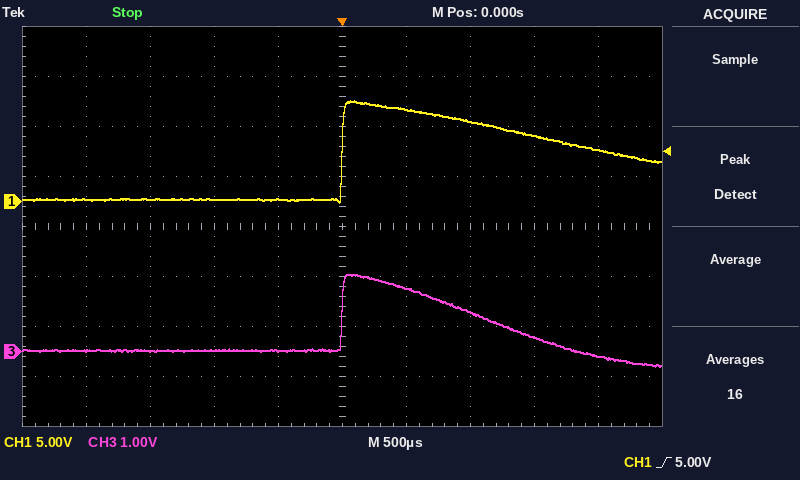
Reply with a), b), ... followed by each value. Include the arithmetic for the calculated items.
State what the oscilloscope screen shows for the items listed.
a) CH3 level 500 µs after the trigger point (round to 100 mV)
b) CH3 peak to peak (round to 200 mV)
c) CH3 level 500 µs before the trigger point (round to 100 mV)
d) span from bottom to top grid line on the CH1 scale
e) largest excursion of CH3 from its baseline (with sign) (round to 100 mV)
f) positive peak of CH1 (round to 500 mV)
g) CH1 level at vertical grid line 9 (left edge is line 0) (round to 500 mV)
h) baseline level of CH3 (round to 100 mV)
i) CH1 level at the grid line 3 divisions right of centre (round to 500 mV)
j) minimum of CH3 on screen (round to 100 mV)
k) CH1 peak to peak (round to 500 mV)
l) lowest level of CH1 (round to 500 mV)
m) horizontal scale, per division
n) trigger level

a) 1.3 V
b) 1.8 V
c) 0.0 V
d) 40 V
e) +1.5 V
f) 10.0 V
g) 5.0 V
h) 0.0 V
i) 6.5 V
j) -300 mV
k) 10.0 V − (0.0 V) = 10.0 V
l) 0.0 V
m) 500 µs
n) 5.00 V
